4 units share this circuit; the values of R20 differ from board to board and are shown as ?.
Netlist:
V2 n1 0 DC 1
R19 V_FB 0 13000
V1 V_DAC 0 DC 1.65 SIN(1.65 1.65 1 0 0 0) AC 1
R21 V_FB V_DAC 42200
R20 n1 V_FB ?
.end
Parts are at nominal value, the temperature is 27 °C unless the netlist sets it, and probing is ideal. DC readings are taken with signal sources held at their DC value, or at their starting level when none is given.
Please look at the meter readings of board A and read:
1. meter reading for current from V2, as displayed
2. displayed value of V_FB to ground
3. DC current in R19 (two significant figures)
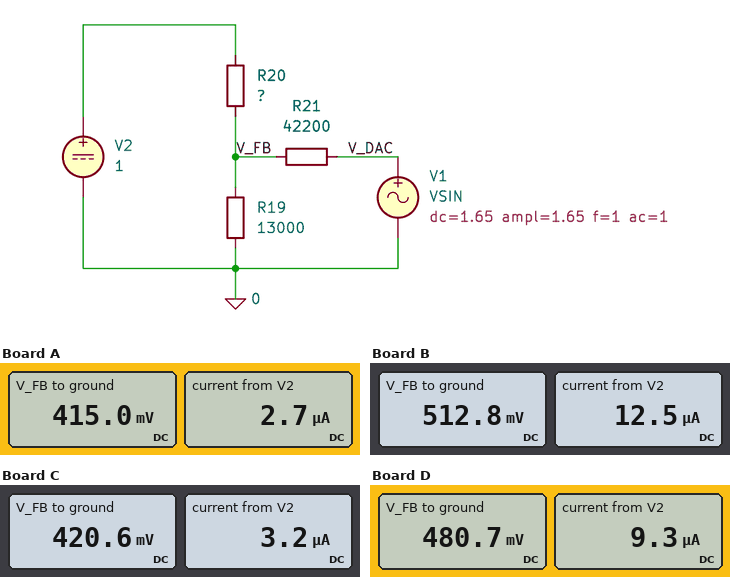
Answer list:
2.7 µA
415.0 mV
32 µA
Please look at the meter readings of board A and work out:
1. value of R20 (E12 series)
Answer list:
220 kΩ
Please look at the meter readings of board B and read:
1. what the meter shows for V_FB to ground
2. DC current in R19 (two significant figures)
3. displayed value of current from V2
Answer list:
512.8 mV
39 µA
12.5 µA
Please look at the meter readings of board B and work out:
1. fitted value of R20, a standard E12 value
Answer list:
39 kΩ
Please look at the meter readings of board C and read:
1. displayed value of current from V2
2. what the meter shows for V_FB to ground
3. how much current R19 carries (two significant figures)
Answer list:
3.2 µA
420.6 mV
32 µA
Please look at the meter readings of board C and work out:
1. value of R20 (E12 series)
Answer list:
180 kΩ
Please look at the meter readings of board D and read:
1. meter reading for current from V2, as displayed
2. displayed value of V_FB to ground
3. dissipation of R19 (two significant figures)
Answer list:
9.3 µA
480.7 mV
18 µW
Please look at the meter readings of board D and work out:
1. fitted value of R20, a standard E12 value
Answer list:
56 kΩ
